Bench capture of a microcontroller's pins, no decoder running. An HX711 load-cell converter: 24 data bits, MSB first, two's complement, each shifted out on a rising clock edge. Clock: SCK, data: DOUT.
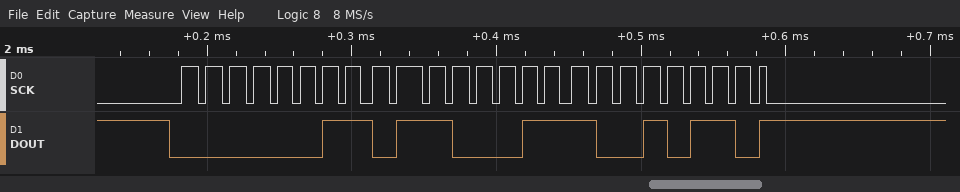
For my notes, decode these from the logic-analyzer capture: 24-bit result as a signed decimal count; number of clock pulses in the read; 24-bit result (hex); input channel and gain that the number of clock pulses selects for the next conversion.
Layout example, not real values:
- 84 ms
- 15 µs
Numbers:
- 222102
- 25
- 0x036396
- channel A, gain 128
